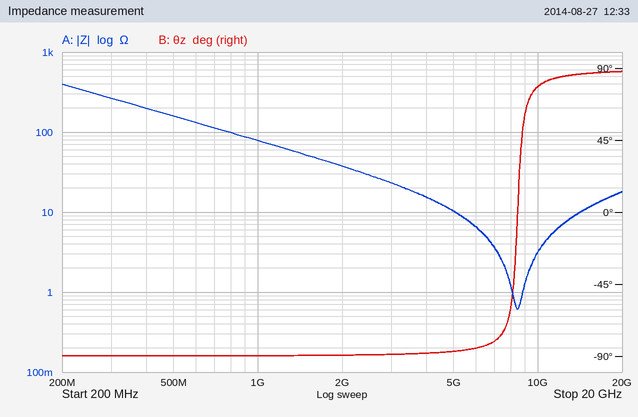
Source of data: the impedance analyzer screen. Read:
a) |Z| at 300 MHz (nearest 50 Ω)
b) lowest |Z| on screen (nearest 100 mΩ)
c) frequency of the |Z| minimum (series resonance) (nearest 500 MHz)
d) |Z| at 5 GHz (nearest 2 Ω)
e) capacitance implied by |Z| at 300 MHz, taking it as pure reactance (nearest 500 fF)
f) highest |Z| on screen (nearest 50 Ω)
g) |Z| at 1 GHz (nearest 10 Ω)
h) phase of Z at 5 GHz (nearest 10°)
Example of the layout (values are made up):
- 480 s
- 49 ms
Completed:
- 250 Ω
- 600 mΩ
- 8.5 GHz
- 10 Ω
- 2.0 pF
- 400 Ω
- 80 Ω
- -90°
